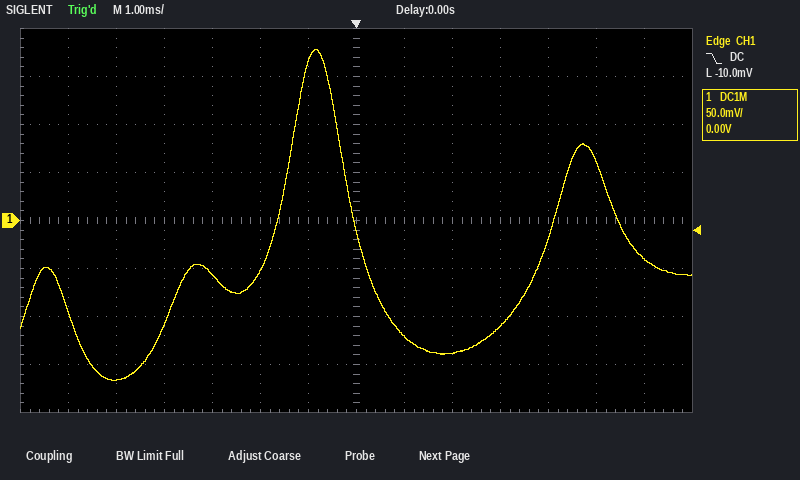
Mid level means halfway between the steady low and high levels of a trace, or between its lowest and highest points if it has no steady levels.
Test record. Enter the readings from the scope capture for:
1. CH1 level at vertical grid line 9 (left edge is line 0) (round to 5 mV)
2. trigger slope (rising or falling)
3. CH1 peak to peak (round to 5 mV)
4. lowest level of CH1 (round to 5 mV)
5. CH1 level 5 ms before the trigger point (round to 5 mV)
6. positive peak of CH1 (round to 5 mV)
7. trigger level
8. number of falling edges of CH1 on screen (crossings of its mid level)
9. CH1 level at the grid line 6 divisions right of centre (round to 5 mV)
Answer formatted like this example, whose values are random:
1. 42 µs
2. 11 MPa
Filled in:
1. -140 mV
2. falling
3. 345 mV
4. -165 mV
5. -165 mV
6. 180 mV
7. -10.0 mV
8. 2
9. -40 mV
